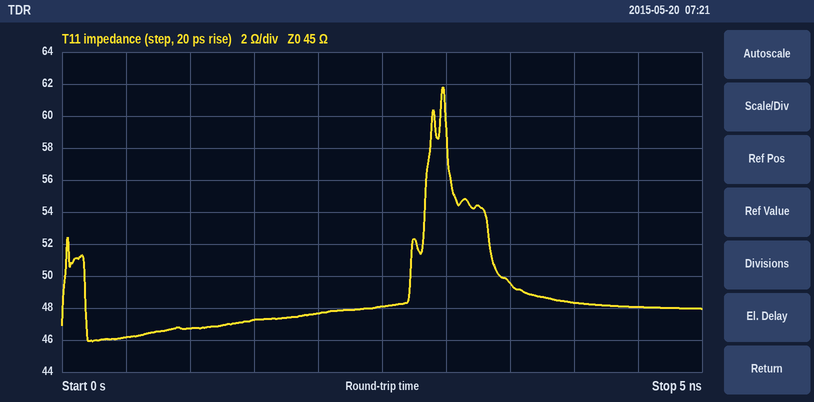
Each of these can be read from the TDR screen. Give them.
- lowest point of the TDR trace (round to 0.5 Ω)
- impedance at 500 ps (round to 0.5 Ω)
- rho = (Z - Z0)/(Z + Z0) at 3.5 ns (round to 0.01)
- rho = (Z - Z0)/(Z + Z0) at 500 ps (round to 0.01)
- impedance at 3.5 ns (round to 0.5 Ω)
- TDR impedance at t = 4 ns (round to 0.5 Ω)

46.0 Ω
46.0 Ω
+0.05
+0.01
49.5 Ω
48.5 Ω
